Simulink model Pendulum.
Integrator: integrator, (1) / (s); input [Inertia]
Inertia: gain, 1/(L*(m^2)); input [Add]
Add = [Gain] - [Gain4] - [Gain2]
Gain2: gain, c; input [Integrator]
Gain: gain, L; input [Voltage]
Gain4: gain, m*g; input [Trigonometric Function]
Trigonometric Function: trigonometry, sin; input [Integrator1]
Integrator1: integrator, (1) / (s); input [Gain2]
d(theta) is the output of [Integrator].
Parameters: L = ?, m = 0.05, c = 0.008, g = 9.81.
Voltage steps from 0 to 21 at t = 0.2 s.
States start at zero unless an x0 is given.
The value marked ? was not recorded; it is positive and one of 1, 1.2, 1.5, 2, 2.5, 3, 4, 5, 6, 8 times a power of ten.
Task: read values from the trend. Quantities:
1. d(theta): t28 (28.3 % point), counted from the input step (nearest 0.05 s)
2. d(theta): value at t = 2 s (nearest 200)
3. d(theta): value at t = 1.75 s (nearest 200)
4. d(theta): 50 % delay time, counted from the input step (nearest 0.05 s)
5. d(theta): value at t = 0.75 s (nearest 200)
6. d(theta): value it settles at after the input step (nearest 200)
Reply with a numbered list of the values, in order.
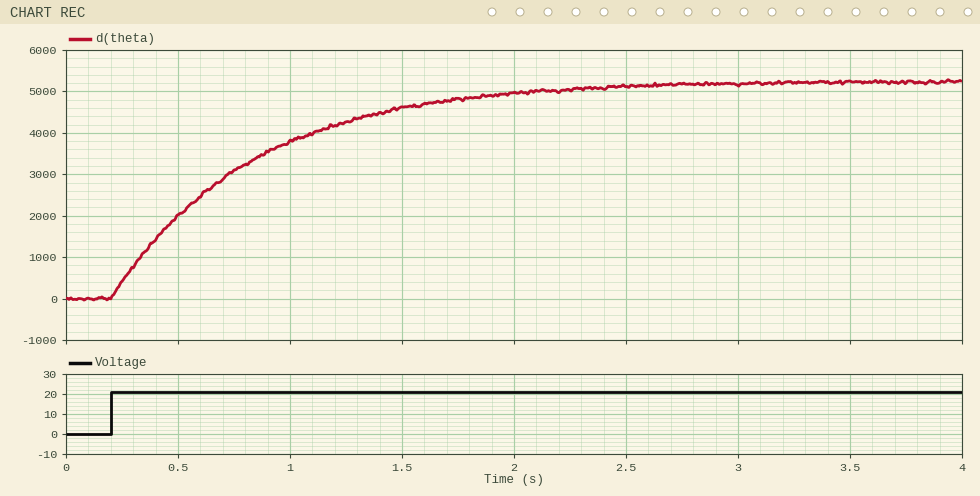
1. 0.20 s
2. 5000
3. 4800
4. 0.45 s
5. 3000
6. 5200
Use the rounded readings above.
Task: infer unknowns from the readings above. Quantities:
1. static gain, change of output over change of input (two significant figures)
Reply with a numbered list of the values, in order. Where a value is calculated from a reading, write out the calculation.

1. (5200 - 0) / (21 - 0) = 250
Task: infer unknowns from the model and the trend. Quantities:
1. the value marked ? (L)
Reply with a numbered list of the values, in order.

1. 2
